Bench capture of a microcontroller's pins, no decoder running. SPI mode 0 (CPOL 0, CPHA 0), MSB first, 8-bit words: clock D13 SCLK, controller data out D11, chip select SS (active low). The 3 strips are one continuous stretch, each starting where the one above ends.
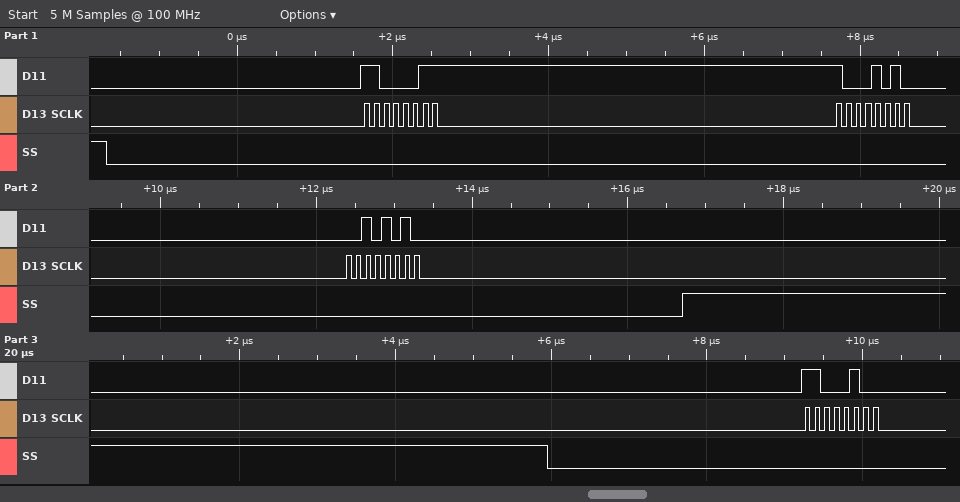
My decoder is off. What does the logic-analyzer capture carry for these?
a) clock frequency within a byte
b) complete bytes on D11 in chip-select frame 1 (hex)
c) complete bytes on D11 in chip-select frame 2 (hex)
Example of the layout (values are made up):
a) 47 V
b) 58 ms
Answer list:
a) 8 MHz
b) C3 8A 2A
c) C4
